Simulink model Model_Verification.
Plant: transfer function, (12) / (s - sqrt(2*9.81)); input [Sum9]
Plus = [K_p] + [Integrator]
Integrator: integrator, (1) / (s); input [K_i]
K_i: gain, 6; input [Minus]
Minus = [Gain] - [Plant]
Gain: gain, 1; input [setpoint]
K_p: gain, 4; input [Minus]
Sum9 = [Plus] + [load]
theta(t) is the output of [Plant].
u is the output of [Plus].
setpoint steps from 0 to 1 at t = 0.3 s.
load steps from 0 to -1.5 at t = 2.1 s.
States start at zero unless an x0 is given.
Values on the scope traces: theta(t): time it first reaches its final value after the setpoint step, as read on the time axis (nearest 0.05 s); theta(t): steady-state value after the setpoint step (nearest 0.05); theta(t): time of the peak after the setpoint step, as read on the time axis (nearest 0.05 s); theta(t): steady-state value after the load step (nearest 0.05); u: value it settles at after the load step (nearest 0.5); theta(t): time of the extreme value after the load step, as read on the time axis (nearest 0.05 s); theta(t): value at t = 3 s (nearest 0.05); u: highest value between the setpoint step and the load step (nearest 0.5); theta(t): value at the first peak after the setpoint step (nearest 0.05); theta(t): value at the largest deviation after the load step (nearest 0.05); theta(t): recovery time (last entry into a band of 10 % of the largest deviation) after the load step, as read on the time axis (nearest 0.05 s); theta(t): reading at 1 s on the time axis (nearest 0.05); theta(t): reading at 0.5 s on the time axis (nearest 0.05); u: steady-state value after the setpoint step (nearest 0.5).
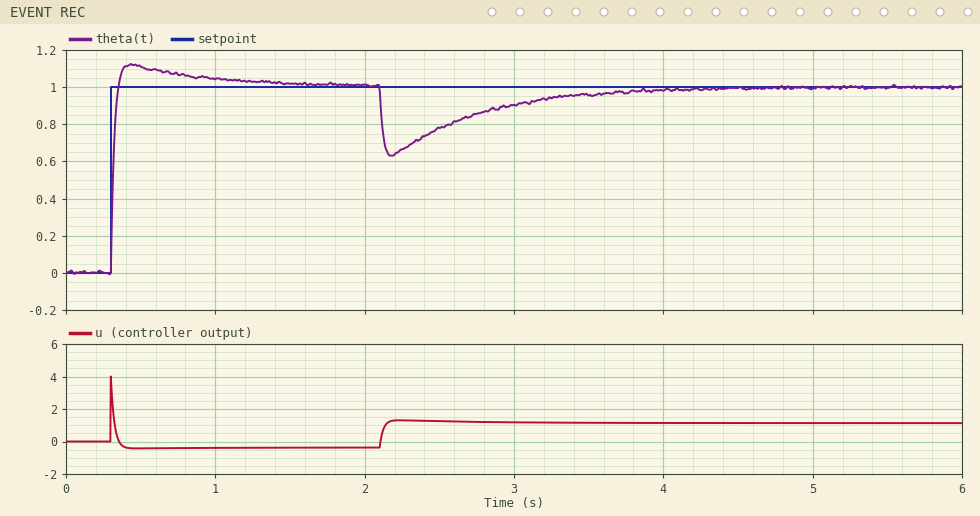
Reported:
0.35 s
1.00
0.45 s
1.00
1.0
2.20 s
0.90
4.0
1.10
0.65
3.55 s
1.05
1.10
-0.5
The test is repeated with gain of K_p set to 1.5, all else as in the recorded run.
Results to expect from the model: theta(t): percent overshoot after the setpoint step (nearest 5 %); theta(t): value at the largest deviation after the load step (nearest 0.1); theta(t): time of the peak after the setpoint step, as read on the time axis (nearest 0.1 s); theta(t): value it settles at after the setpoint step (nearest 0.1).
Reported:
35 %
0.1
0.5 s
1.0
